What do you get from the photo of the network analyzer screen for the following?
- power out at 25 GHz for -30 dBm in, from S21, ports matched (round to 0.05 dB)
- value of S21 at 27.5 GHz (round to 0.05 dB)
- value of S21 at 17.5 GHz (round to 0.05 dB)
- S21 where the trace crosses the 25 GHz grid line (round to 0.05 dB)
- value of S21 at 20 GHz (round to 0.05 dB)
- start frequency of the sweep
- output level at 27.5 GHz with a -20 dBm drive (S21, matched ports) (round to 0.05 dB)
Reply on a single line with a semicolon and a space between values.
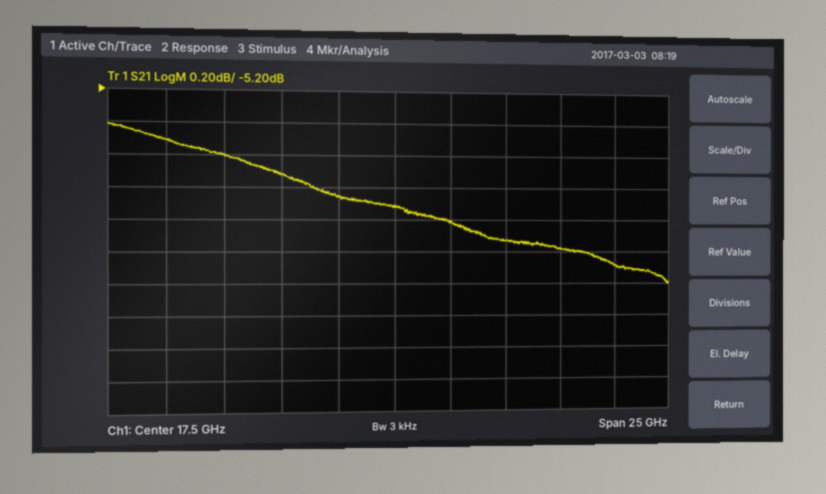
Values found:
-36.20 dBm; -6.30 dB; -5.90 dB; -6.20 dB; -6.00 dB; 5 GHz; -26.30 dBm
